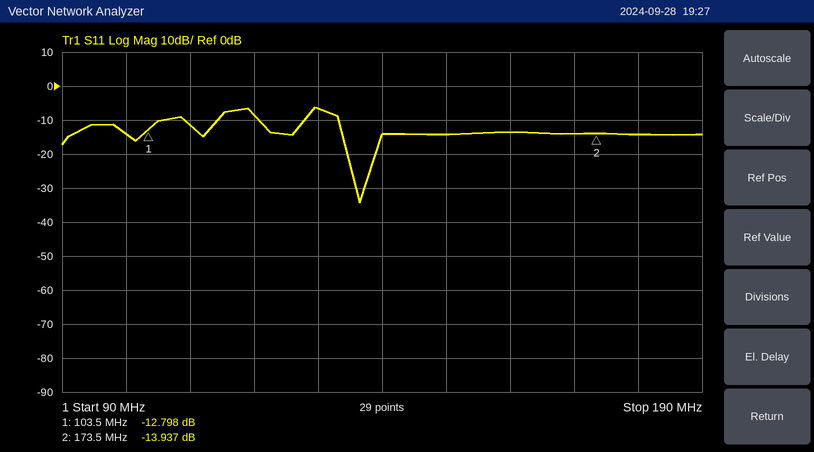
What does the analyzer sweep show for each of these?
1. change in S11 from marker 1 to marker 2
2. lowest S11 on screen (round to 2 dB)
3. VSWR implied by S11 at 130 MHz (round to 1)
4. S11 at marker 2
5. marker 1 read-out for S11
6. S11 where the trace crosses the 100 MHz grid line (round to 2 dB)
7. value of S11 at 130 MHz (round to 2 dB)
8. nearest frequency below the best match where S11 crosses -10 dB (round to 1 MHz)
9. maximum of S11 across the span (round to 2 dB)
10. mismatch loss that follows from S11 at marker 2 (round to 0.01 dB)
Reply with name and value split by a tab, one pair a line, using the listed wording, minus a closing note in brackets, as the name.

change in S11 from marker 1 to marker 2	-1.139 dB
lowest S11 on screen	-34 dB
VSWR implied by S11 at 130 MHz	3
S11 at marker 2	-13.937 dB
marker 1 read-out for S11	-12.798 dB
S11 where the trace crosses the 100 MHz grid line	-14 dB
value of S11 at 130 MHz	-6 dB
nearest frequency below the best match where S11 crosses -10 dB	133 MHz
maximum of S11 across the span	-6 dB
mismatch loss that follows from S11 at marker 2	0.18 dB
